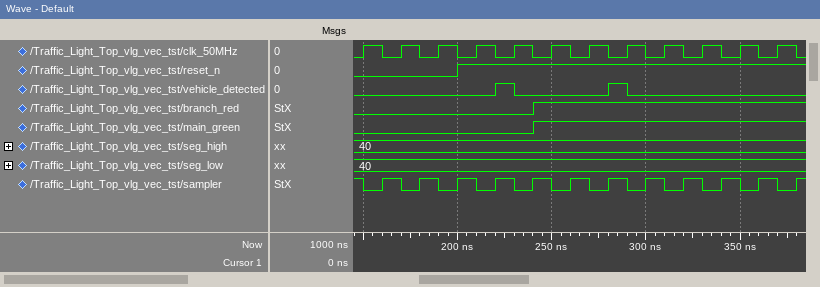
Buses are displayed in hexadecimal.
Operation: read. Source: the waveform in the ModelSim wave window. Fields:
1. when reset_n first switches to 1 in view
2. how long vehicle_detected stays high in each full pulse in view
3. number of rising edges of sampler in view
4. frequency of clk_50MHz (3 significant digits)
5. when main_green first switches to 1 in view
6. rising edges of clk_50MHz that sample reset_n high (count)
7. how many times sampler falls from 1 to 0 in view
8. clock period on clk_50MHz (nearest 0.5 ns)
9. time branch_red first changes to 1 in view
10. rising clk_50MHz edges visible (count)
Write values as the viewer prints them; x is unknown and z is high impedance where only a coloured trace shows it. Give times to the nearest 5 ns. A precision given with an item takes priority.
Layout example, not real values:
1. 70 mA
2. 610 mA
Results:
1. 200 ns
2. 10 ns, 10 ns
3. 12
4. 50.0 MHz
5. 240 ns
6. 9
7. 12
8. 20 ns
9. 240 ns
10. 12
